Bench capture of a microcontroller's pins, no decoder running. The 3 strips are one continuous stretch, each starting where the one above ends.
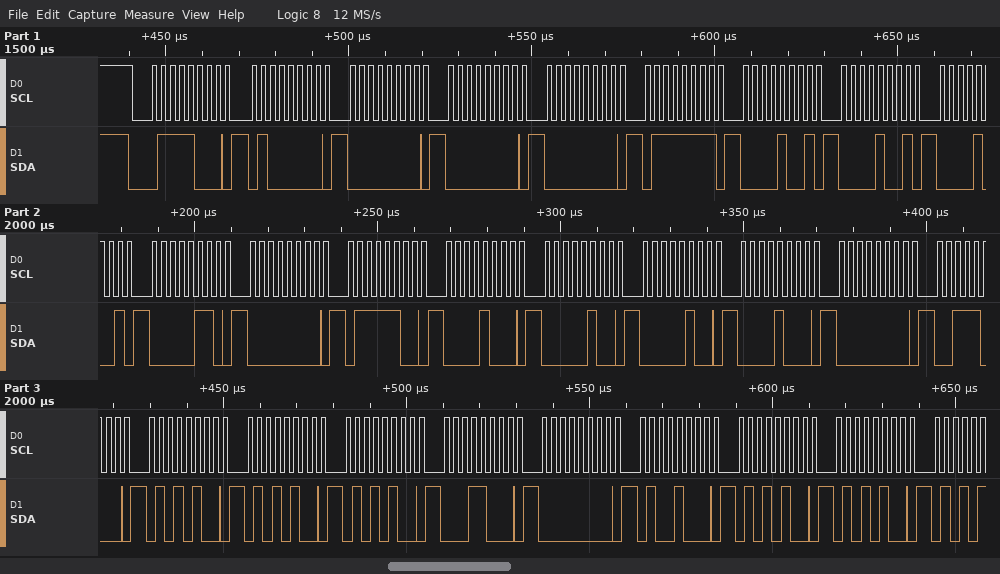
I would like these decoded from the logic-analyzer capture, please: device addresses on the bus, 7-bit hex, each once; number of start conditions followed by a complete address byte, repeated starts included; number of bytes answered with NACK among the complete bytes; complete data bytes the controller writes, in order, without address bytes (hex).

0x3C
1
0
40 00 00 00 7F 09 09 09 06 00 7C 08 04 04 08 00 38 54 54 54 18 00 48 54 54
